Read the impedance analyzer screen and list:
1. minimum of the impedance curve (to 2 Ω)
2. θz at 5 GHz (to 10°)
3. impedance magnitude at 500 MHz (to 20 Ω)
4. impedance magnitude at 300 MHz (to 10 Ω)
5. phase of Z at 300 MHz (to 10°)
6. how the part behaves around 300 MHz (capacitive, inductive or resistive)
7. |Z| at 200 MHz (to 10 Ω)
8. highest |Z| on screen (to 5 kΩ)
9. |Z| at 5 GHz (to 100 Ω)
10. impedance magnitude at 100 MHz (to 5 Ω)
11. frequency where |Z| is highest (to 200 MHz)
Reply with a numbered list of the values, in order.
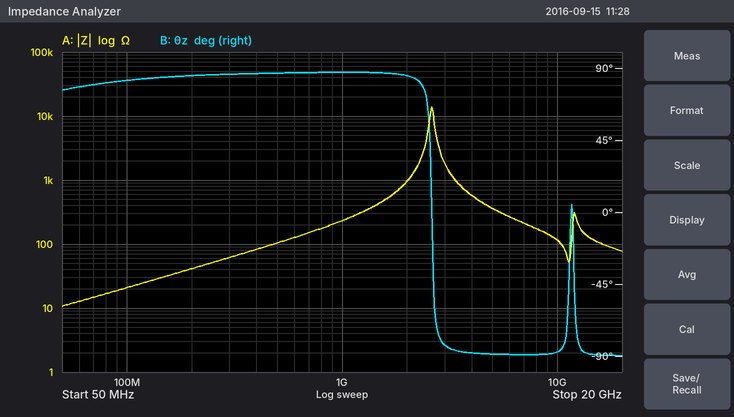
1. 10 Ω
2. -90°
3. 100 Ω
4. 60 Ω
5. 90°
6. inductive
7. 40 Ω
8. 15 kΩ
9. 400 Ω
10. 20 Ω
11. 2.6 GHz
